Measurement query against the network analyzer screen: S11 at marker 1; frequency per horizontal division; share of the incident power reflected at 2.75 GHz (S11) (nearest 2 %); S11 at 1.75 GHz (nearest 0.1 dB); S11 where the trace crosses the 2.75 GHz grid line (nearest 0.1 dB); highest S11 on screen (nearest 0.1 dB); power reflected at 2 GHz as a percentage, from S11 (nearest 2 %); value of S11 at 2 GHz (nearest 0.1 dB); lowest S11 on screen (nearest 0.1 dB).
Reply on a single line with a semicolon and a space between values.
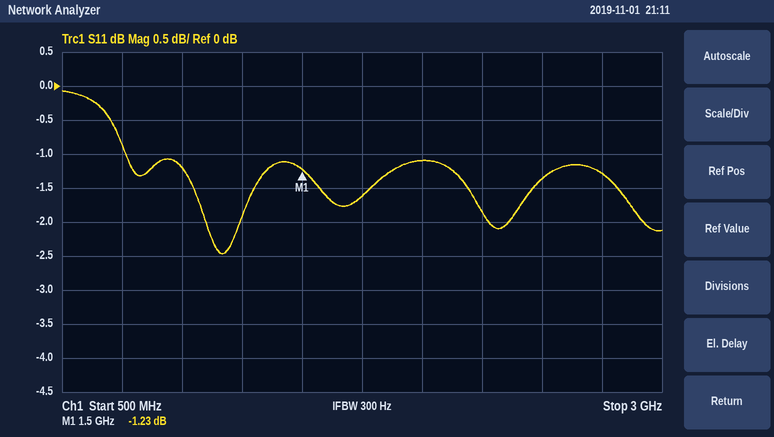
-1.23 dB; 250 MHz; 74 %; -1.6 dB; -1.3 dB; -0.1 dB; 78 %; -1.1 dB; -2.5 dB
